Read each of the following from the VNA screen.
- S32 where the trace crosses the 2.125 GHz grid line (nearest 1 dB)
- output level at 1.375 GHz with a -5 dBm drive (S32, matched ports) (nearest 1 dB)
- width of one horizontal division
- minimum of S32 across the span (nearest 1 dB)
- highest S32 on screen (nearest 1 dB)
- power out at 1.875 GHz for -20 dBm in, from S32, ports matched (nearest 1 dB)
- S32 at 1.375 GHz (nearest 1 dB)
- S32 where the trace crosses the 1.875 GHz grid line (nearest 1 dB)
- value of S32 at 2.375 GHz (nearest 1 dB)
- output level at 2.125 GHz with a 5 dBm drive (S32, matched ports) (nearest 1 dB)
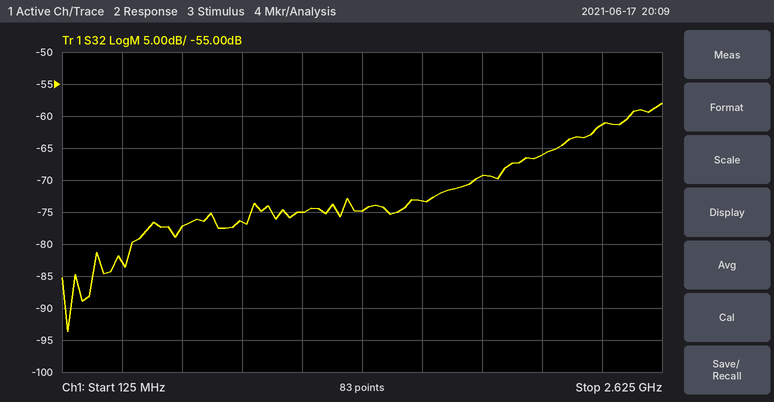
-66 dB
-80 dBm
250 MHz
-94 dB
-58 dB
-89 dBm
-75 dB
-69 dB
-61 dB
-61 dBm
